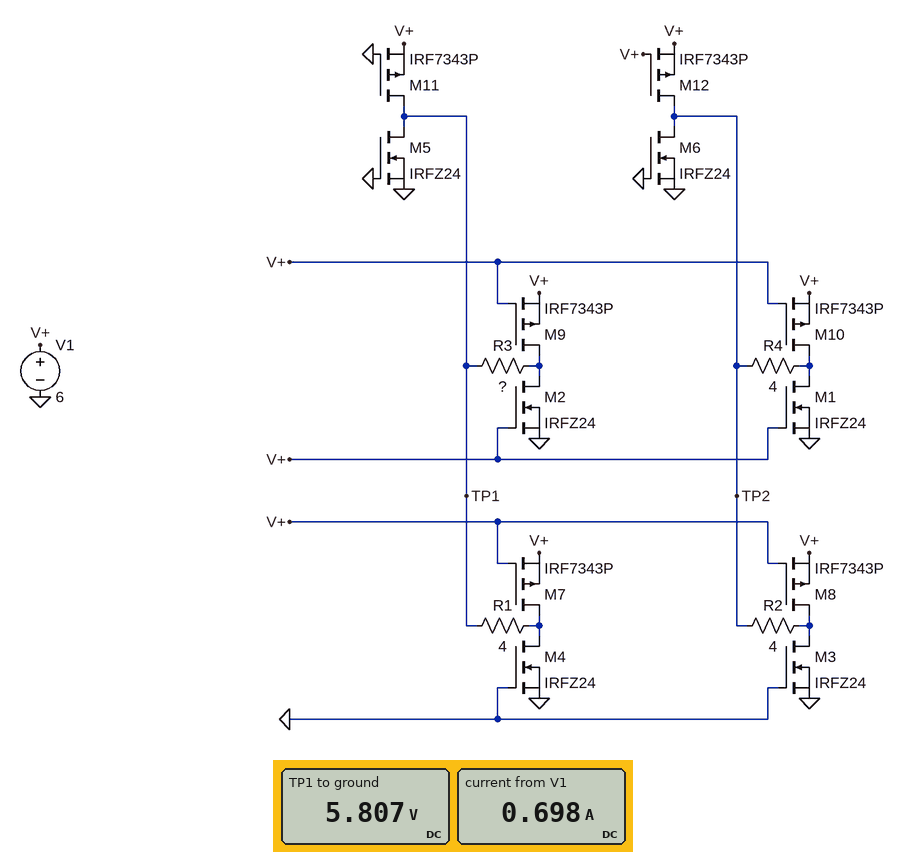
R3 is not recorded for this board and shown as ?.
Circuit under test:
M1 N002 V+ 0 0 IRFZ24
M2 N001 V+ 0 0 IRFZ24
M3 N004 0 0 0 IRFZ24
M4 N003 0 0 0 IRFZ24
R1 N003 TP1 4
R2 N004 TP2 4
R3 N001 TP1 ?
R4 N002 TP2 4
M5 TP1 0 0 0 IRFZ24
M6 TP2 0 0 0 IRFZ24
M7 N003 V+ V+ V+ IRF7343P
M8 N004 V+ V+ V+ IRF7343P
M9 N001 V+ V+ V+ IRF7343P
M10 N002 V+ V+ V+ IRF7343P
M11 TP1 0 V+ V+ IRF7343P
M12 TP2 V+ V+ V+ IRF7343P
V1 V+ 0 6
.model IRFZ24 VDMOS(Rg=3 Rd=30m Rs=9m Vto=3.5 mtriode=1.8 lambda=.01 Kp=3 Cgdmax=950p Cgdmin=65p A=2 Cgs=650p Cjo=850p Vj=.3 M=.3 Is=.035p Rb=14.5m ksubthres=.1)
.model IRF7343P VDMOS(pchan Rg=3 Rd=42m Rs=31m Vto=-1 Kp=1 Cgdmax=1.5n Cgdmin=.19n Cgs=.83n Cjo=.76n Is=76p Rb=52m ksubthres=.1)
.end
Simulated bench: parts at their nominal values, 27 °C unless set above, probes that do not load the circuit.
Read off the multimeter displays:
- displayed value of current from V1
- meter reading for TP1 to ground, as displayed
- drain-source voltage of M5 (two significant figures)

0.698 A
5.807 V
5.8 V
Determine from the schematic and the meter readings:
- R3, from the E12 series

8.2 Ω
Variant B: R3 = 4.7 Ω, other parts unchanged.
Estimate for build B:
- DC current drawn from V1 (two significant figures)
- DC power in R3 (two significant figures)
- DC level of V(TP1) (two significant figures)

1.2 A
6.5 W
5.7 V
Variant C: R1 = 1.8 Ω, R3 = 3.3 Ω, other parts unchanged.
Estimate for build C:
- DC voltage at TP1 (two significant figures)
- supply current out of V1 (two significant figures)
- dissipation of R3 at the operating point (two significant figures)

5.5 V
1.6 A
8.7 W
